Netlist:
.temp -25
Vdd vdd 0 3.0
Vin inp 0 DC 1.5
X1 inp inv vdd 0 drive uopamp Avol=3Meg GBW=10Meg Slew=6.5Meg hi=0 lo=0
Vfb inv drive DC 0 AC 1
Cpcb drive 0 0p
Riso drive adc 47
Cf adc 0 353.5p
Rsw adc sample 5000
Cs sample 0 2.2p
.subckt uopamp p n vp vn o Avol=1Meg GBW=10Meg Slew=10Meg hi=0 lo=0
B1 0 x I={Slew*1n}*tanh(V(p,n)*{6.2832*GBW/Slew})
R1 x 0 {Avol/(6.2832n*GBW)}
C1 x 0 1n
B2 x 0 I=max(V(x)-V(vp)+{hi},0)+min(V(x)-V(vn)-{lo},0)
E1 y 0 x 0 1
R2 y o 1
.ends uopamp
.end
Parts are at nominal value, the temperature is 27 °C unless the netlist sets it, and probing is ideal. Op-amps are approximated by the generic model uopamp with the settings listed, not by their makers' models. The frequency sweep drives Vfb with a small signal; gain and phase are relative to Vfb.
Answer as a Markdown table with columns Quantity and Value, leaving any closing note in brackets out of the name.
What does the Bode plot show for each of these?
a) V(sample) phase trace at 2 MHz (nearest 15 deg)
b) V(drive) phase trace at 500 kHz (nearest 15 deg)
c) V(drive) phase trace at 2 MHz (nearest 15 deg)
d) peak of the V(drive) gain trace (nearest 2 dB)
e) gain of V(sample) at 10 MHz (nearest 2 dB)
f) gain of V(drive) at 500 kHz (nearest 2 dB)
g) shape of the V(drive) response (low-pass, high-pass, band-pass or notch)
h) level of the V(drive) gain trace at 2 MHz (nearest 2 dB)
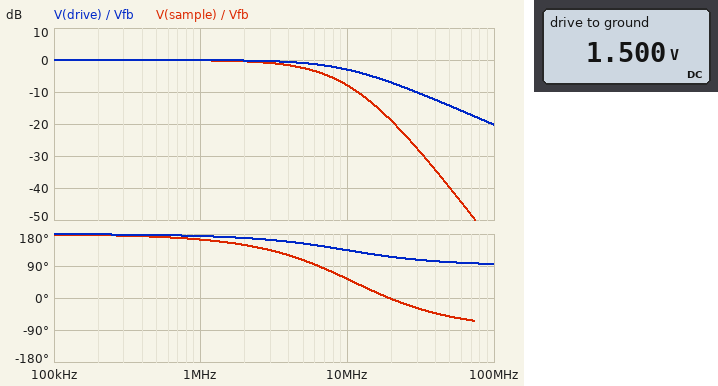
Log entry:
| Quantity | Value |
|---|---|
| V(sample) phase trace at 2 MHz | 150 deg |
| V(drive) phase trace at 500 kHz | 180 deg |
| V(drive) phase trace at 2 MHz | 165 deg |
| peak of the V(drive) gain trace | 0 dB |
| gain of V(sample) at 10 MHz | -8 dB |
| gain of V(drive) at 500 kHz | 0 dB |
| shape of the V(drive) response | low-pass |
| level of the V(drive) gain trace at 2 MHz | 0 dB |
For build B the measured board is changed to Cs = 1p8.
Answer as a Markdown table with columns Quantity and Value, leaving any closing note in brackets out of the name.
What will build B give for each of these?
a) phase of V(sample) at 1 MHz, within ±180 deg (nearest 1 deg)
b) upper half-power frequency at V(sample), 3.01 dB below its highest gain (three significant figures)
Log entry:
| Quantity | Value |
|---|---|
| phase of V(sample) at 1 MHz, within ±180 deg | 165 deg |
| upper half-power frequency at V(sample), 3.01 dB below its highest gain | 5.75 MHz |
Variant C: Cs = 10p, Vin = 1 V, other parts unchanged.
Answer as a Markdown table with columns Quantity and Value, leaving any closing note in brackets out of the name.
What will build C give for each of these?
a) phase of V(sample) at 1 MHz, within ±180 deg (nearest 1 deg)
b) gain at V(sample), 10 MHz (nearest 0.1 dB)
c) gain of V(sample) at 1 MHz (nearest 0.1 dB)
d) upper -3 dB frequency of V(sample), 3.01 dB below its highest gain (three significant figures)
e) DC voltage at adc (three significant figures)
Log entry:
| Quantity | Value |
|---|---|
| phase of V(sample) at 1 MHz, within ±180 deg | 151 deg |
| gain at V(sample), 10 MHz | -16.6 dB |
| gain of V(sample) at 1 MHz | -0.5 dB |
| upper -3 dB frequency of V(sample), 3.01 dB below its highest gain | 2.69 MHz |
| DC voltage at adc | 1.00 V |
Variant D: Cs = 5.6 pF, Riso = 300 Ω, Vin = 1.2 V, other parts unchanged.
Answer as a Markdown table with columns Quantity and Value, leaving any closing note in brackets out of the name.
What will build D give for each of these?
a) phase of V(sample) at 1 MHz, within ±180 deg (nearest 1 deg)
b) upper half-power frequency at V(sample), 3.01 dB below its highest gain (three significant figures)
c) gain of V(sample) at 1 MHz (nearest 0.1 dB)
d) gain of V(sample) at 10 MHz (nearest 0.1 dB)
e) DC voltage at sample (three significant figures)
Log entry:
| Quantity | Value |
|---|---|
| phase of V(sample) at 1 MHz, within ±180 deg | 130 deg |
| upper half-power frequency at V(sample), 3.01 dB below its highest gain | 1.36 MHz |
| gain of V(sample) at 1 MHz | -1.8 dB |
| gain of V(sample) at 10 MHz | -25.8 dB |
| DC voltage at sample | 1.20 V |
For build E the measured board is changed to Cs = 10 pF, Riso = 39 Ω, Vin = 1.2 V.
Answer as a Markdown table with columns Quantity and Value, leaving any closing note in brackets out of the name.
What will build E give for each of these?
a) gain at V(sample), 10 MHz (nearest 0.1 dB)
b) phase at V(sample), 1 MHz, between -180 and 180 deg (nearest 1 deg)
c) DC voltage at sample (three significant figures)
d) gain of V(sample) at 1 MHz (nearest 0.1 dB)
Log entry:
| Quantity | Value |
|---|---|
| gain at V(sample), 10 MHz | -15.8 dB |
| phase at V(sample), 1 MHz, between -180 and 180 deg | 152 deg |
| DC voltage at sample | 1.20 V |
| gain of V(sample) at 1 MHz | -0.5 dB |
